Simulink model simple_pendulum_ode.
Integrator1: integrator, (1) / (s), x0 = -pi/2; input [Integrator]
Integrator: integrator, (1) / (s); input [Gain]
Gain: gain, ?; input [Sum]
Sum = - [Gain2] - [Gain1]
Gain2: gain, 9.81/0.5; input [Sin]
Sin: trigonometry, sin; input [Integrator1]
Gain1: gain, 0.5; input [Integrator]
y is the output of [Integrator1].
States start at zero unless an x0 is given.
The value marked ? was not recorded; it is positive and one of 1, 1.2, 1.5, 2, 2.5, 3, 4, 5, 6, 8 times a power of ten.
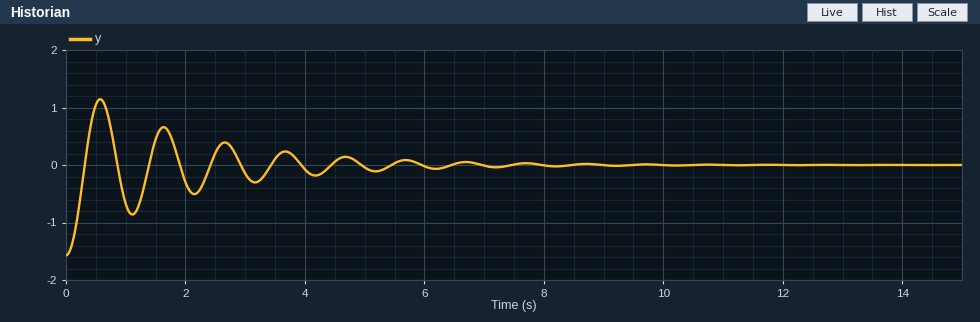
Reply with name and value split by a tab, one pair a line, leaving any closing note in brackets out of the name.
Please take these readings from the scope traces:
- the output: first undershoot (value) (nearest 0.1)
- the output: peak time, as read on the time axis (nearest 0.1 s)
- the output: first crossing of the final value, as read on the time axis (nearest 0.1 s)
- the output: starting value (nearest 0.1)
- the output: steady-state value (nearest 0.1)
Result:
the output: first undershoot (value)	-0.9
the output: peak time, as read on the time axis	0.6 s
the output: first crossing of the final value, as read on the time axis	0.3 s
the output: starting value	-1.6
the output: steady-state value	0.0
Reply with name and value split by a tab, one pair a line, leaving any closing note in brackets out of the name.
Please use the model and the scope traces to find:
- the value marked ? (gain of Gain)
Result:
the value marked ?	2
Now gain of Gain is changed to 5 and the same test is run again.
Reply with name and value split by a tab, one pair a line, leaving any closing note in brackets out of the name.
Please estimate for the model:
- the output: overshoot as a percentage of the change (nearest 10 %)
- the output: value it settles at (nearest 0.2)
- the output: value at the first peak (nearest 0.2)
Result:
the output: overshoot as a percentage of the change	60 %
the output: value it settles at	0.0
the output: value at the first peak	1.0
